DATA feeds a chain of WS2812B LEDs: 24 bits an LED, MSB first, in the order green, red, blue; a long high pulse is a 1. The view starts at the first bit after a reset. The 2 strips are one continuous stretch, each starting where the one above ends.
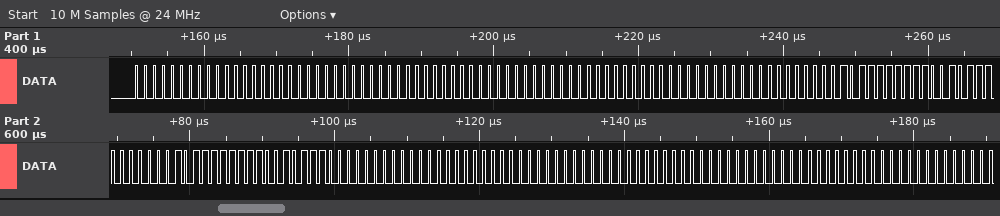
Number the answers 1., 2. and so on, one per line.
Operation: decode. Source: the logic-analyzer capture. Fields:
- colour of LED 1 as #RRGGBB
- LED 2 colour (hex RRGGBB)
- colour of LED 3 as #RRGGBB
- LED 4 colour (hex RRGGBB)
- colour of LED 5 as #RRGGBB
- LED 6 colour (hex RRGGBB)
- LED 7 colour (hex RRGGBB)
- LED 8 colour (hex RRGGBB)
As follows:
1. #000000
2. #000000
3. #000000
4. #FF022E
5. #FF022E
6. #000000
7. #000000
8. #000000
